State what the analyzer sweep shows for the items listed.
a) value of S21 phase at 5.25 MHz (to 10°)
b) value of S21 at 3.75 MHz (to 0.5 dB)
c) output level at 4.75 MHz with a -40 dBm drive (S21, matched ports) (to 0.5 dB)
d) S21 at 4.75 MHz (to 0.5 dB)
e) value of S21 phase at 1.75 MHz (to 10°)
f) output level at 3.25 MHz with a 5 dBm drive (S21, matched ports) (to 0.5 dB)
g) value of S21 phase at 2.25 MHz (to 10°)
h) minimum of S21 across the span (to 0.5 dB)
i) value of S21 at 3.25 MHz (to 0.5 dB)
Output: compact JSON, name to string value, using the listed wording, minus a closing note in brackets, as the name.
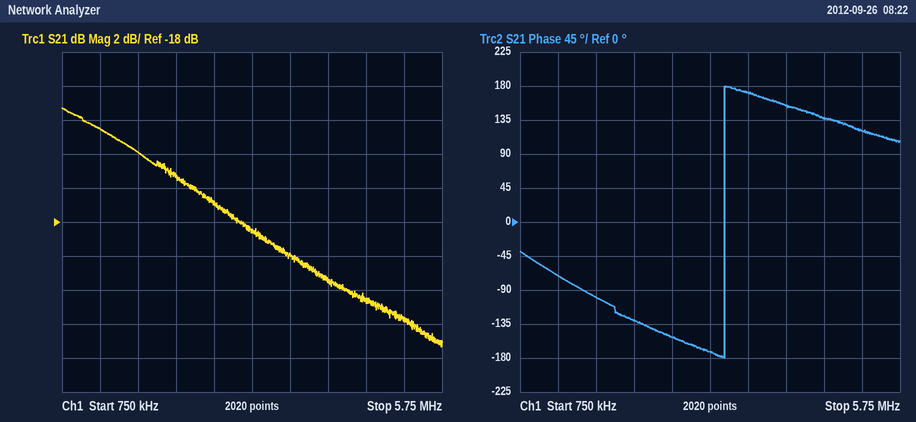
{"value of S21 phase at 5.25 MHz": "120°", "value of S21 at 3.75 MHz": "-20.0 dB", "output level at 4.75 MHz with a -40 dBm drive (S21, matched ports)": "-62.5 dBm", "S21 at 4.75 MHz": "-22.5 dB", "value of S21 phase at 1.75 MHz": "-100°", "output level at 3.25 MHz with a 5 dBm drive (S21, matched ports)": "-13.5 dBm", "value of S21 phase at 2.25 MHz": "-130°", "minimum of S21 across the span": "-25.5 dB", "value of S21 at 3.25 MHz": "-18.5 dB"}
